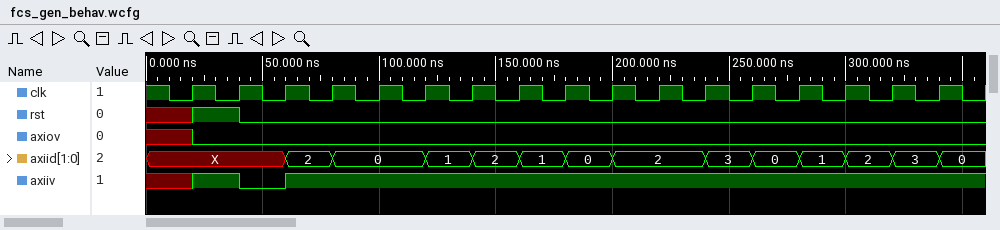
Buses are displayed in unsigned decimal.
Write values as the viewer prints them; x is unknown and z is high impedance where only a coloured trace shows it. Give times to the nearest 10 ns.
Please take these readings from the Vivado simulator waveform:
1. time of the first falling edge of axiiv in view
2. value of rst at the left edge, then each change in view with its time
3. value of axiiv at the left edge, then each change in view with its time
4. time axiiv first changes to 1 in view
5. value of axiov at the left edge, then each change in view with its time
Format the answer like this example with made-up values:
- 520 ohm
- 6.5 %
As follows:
- 40 ns
- x, 1 at 20 ns, 0 at 40 ns
- x, 1 at 20 ns, 0 at 40 ns, 1 at 60 ns
- 20 ns
- x, 0 at 20 ns
